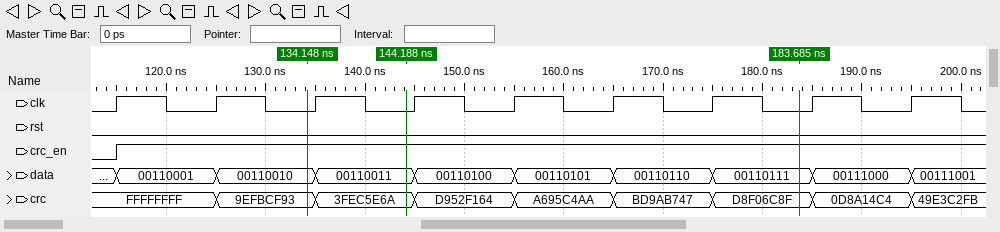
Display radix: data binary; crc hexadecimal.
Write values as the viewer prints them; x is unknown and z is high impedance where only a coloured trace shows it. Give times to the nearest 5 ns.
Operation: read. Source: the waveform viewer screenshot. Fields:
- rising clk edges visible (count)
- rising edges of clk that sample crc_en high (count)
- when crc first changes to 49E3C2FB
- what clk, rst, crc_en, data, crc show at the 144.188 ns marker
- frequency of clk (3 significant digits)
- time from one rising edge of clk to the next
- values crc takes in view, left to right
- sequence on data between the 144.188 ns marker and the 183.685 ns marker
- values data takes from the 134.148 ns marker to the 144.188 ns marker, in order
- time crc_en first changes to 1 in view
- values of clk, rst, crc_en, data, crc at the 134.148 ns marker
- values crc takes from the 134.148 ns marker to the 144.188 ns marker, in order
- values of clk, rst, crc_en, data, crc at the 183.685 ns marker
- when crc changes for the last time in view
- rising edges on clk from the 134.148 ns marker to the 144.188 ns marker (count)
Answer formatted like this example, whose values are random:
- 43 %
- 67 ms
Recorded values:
- 9
- 8
- 195 ns
- clk=0, rst=0, crc_en=1, data=00110011, crc=3FEC5E6A
- 100 MHz
- 10 ns
- FFFFFFFF, 9EFBCF93, 3FEC5E6A, D952F164, A695C4AA, BD9AB747, D8F06C8F, 0D8A14C4, 49E3C2FB
- 00110011, 00110100, 00110101, 00110110, 00110111
- 00110010, 00110011
- 115 ns
- clk=0, rst=0, crc_en=1, data=00110010, crc=9EFBCF93
- 9EFBCF93, 3FEC5E6A
- clk=0, rst=0, crc_en=1, data=00110111, crc=D8F06C8F
- 195 ns
- 1
